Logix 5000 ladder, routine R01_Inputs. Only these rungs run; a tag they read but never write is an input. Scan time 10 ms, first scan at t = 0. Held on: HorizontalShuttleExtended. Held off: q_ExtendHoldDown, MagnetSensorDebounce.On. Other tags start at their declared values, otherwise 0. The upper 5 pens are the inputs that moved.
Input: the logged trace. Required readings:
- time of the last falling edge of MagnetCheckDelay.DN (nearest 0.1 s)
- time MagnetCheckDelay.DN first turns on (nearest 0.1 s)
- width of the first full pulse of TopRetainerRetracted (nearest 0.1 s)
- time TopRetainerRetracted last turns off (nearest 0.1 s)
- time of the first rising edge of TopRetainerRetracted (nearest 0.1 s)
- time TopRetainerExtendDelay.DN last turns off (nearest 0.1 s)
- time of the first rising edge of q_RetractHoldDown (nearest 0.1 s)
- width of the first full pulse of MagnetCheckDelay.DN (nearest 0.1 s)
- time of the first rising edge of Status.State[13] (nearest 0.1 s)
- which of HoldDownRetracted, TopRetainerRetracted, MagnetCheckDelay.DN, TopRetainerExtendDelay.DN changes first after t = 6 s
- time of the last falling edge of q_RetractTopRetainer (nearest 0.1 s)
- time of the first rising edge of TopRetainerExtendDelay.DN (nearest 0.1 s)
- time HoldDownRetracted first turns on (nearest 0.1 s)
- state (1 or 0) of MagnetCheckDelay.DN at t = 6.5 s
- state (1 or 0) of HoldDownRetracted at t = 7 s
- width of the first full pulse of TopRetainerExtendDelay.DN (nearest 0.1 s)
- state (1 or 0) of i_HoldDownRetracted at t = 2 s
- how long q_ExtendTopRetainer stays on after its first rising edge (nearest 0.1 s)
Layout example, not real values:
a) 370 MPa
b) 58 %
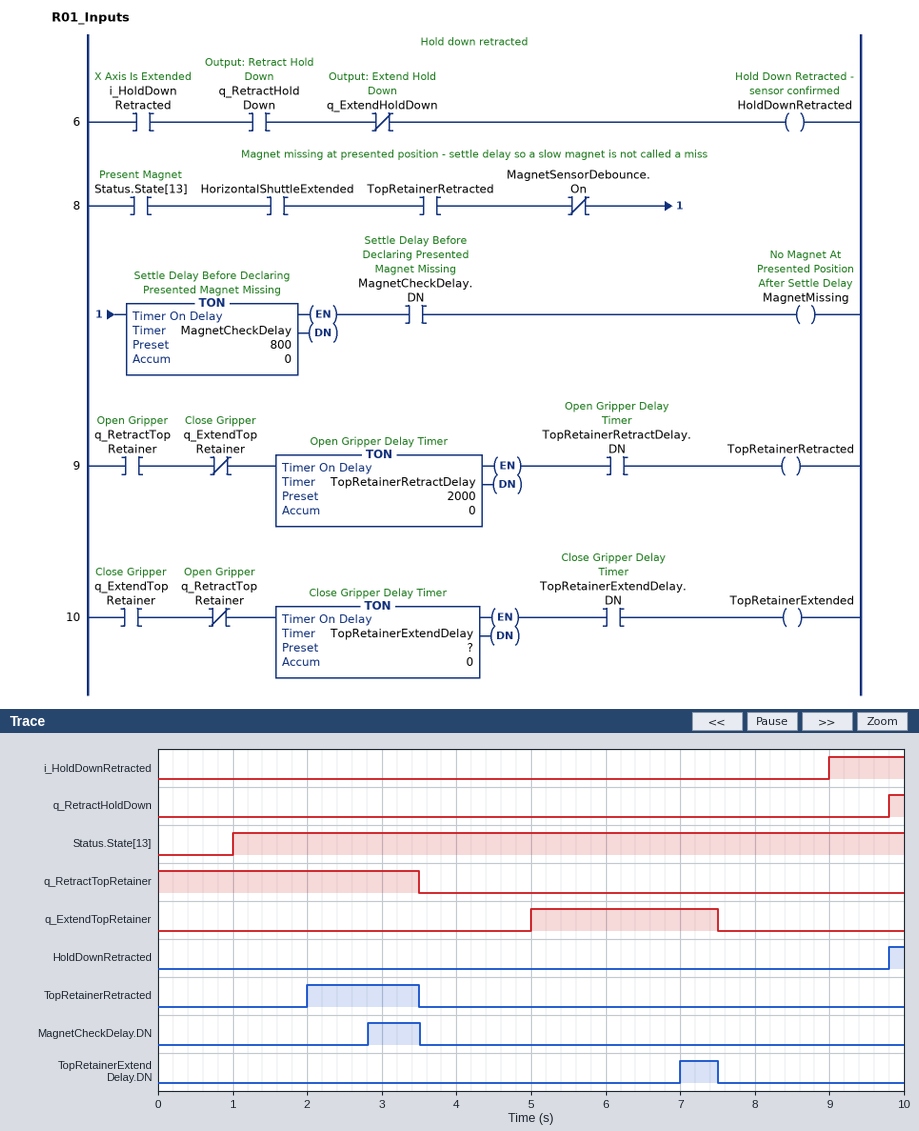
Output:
a) 3.5 s
b) 2.8 s
c) 1.5 s
d) 3.5 s
e) 2.0 s
f) 7.5 s
g) 9.8 s
h) 0.7 s
i) 1.0 s
j) TopRetainerExtendDelay.DN
k) 3.5 s
l) 7.0 s
m) 9.8 s
n) 0
o) 0
p) 0.5 s
q) 0
r) 2.5 s
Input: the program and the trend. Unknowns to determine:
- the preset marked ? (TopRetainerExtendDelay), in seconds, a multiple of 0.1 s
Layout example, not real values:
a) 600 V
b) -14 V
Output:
a) 2.0 s
